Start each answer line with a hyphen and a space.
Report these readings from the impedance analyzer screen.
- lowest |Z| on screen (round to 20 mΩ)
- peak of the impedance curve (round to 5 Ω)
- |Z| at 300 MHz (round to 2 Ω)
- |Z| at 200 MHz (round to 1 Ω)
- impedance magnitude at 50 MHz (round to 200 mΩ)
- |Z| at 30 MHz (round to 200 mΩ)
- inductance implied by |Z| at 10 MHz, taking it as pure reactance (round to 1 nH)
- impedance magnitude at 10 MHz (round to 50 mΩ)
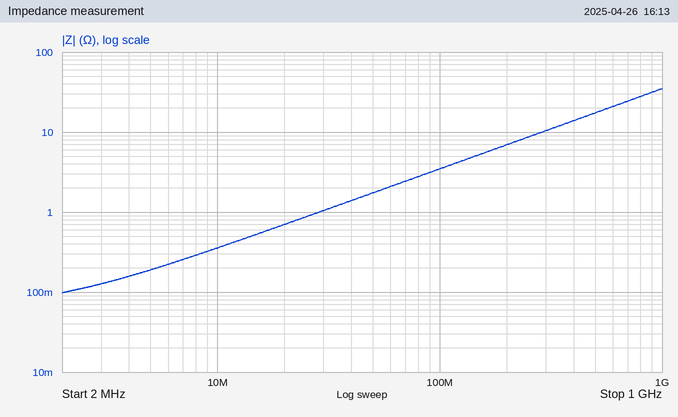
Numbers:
- 100 mΩ
- 35 Ω
- 10 Ω
- 7 Ω
- 1.8 Ω
- 1.0 Ω
- 6 nH
- 350 mΩ
